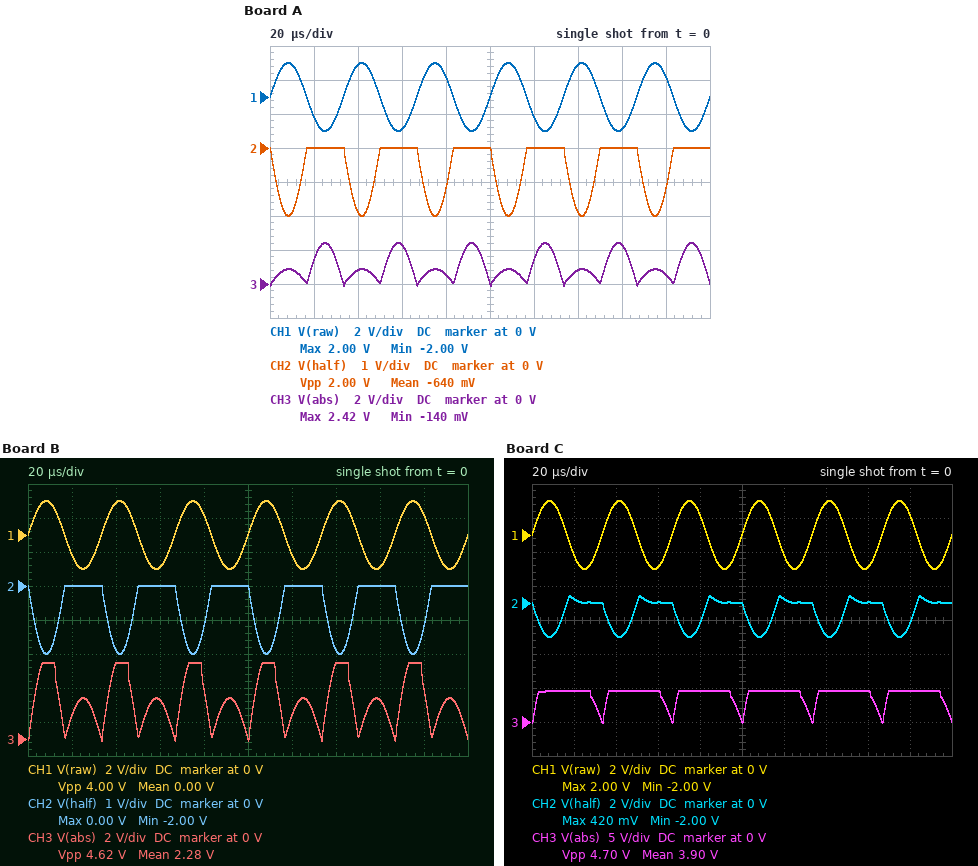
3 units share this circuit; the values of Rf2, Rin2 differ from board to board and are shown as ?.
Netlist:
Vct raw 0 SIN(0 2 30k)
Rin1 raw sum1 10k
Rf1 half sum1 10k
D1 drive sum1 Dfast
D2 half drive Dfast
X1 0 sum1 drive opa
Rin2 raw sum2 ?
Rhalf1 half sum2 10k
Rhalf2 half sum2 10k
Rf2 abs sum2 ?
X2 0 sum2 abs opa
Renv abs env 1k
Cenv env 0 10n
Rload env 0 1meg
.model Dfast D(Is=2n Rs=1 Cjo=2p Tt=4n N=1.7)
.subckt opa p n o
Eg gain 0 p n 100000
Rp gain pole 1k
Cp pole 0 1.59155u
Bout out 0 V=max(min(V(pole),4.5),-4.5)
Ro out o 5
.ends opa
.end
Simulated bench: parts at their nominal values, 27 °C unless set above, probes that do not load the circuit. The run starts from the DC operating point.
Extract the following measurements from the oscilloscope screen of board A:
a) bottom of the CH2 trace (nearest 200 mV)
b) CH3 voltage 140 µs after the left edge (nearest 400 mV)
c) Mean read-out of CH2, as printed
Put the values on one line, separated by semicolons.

-2.0 V; 800 mV; -640 mV
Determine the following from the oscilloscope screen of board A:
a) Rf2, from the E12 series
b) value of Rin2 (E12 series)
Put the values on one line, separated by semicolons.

8.2 kΩ; 6.8 kΩ
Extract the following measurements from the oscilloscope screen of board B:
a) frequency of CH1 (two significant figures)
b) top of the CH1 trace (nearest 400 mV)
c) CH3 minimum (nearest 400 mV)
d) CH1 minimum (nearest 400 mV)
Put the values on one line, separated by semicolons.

30 kHz; 2.0 V; 0 V; -2.0 V
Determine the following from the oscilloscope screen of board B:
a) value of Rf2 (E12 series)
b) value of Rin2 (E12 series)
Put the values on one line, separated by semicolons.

18 kΩ; 15 kΩ
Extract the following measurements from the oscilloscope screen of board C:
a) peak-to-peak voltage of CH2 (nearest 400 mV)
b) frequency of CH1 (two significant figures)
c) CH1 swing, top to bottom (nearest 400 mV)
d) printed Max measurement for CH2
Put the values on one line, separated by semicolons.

2.4 V; 30 kHz; 4.0 V; 420 mV
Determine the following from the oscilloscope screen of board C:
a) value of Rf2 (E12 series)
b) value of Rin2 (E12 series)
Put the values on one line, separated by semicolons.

33 kΩ; 15 kΩ
